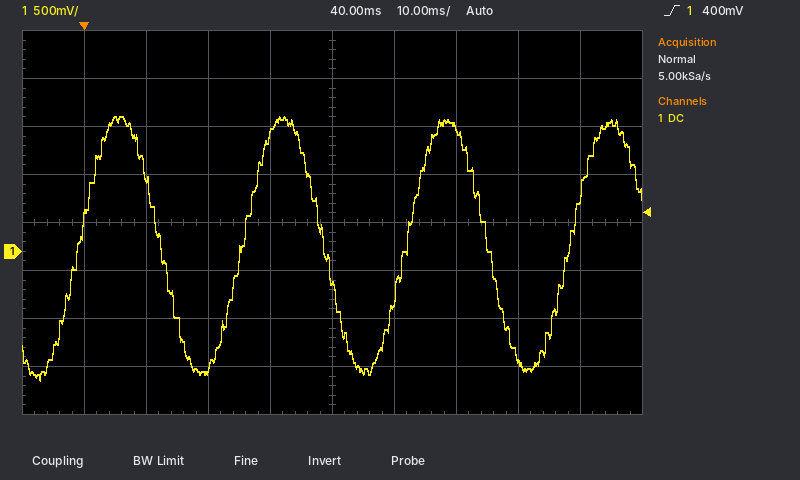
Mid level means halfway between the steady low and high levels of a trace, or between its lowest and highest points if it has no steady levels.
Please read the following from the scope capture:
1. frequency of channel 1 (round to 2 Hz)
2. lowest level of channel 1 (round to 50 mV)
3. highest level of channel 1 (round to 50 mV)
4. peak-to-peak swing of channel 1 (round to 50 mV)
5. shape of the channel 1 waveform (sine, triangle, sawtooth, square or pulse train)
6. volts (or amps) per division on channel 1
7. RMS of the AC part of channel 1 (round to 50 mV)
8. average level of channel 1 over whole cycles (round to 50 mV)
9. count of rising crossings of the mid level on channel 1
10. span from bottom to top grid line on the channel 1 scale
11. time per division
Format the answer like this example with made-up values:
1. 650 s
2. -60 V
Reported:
1. 38 Hz
2. -1.35 V
3. 1.40 V
4. 2.75 V
5. sine
6. 500 mV
7. 950 mV
8. 50 mV
9. 4
10. 4 V
11. 10 ms
